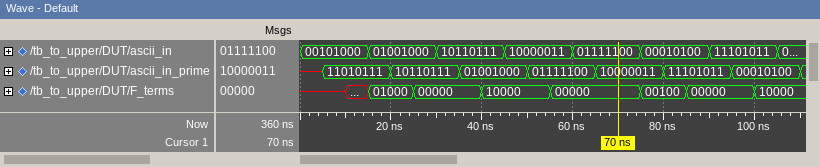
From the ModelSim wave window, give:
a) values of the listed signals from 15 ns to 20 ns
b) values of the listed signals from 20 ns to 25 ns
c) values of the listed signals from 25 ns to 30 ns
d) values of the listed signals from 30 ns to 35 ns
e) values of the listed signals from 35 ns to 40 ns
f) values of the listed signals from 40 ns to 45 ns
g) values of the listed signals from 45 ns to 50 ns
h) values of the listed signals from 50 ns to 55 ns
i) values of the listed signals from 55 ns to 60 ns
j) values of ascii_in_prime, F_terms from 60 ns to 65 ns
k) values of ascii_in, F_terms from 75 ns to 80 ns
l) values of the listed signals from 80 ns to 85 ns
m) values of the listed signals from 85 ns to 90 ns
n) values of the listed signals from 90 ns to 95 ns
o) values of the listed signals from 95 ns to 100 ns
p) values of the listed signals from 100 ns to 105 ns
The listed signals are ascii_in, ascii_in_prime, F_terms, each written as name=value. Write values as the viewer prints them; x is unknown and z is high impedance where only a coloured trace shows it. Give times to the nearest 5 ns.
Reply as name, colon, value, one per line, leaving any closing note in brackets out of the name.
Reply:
values of the listed signals from 15 ns to 20 ns: ascii_in=01001000, ascii_in_prime=11010111, F_terms=01000
values of the listed signals from 20 ns to 25 ns: ascii_in=01001000, ascii_in_prime=10110111, F_terms=01000
values of the listed signals from 25 ns to 30 ns: ascii_in=01001000, ascii_in_prime=10110111, F_terms=00000
values of the listed signals from 30 ns to 35 ns: ascii_in=10110111, ascii_in_prime=10110111, F_terms=00000
values of the listed signals from 35 ns to 40 ns: ascii_in=10110111, ascii_in_prime=01001000, F_terms=00000
values of the listed signals from 40 ns to 45 ns: ascii_in=10110111, ascii_in_prime=01001000, F_terms=10000
values of the listed signals from 45 ns to 50 ns: ascii_in=10000011, ascii_in_prime=01001000, F_terms=10000
values of the listed signals from 50 ns to 55 ns: ascii_in=10000011, ascii_in_prime=01111100, F_terms=10000
values of the listed signals from 55 ns to 60 ns: ascii_in=10000011, ascii_in_prime=01111100, F_terms=00000
values of ascii_in_prime, F_terms from 60 ns to 65 ns: ascii_in_prime=01111100, F_terms=00000
values of ascii_in, F_terms from 75 ns to 80 ns: ascii_in=00010100, F_terms=00100
values of the listed signals from 80 ns to 85 ns: ascii_in=00010100, ascii_in_prime=11101011, F_terms=00100
values of the listed signals from 85 ns to 90 ns: ascii_in=00010100, ascii_in_prime=11101011, F_terms=00000
values of the listed signals from 90 ns to 95 ns: ascii_in=11101011, ascii_in_prime=11101011, F_terms=00000
values of the listed signals from 95 ns to 100 ns: ascii_in=11101011, ascii_in_prime=00010100, F_terms=00000
values of the listed signals from 100 ns to 105 ns: ascii_in=11101011, ascii_in_prime=00010100, F_terms=10000
